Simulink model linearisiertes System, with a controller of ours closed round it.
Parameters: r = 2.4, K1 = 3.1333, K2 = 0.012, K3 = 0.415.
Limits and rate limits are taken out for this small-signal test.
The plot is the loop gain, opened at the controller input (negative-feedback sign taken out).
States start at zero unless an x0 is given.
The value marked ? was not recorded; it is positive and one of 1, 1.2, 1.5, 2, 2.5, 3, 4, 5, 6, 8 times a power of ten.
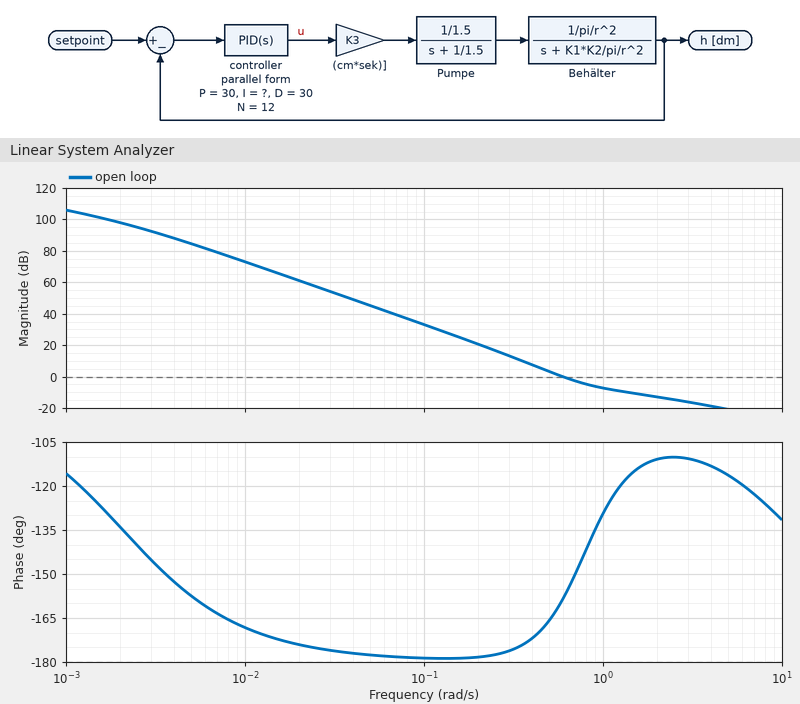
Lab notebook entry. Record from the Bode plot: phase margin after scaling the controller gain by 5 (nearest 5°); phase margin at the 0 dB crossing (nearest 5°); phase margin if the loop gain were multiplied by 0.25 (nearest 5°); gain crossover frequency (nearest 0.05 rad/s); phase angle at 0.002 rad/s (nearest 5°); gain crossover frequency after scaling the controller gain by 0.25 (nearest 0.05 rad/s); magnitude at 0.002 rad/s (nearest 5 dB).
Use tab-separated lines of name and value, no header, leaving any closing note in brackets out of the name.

phase margin after scaling the controller gain by 5	70°
phase margin at the 0 dB crossing	20°
phase margin if the loop gain were multiplied by 0.25	5°
gain crossover frequency	0.60 rad/s
phase angle at 0.002 rad/s	-135°
gain crossover frequency after scaling the controller gain by 0.25	0.30 rad/s
magnitude at 0.002 rad/s	100 dB
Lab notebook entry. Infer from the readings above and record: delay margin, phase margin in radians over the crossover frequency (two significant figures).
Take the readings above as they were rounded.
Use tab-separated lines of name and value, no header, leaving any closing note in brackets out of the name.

delay margin, phase margin in radians over the crossover frequency	0.58 s
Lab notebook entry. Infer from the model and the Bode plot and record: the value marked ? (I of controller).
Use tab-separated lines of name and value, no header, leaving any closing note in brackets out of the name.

the value marked ?	20
